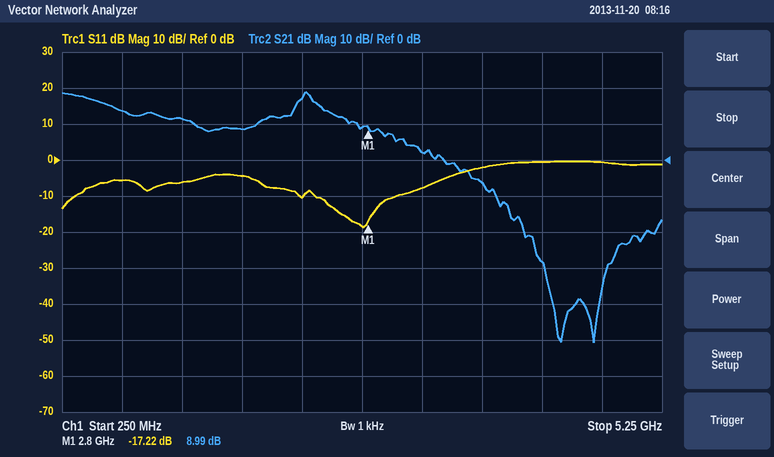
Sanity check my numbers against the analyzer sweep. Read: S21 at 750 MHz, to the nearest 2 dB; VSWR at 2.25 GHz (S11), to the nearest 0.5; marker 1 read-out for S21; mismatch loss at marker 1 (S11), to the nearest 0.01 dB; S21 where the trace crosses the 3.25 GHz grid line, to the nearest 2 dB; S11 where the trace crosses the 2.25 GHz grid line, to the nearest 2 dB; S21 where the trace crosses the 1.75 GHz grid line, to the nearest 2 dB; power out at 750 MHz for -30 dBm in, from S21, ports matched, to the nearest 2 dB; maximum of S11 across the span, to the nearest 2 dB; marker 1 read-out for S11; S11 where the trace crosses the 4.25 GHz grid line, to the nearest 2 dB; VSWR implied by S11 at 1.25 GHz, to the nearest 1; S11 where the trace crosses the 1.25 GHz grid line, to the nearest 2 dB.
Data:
14 dB
2.0
8.99 dB
0.08 dB
2 dB
-10 dB
8 dB
-16 dBm
0 dB
-17.22 dB
0 dB
3
-6 dB
